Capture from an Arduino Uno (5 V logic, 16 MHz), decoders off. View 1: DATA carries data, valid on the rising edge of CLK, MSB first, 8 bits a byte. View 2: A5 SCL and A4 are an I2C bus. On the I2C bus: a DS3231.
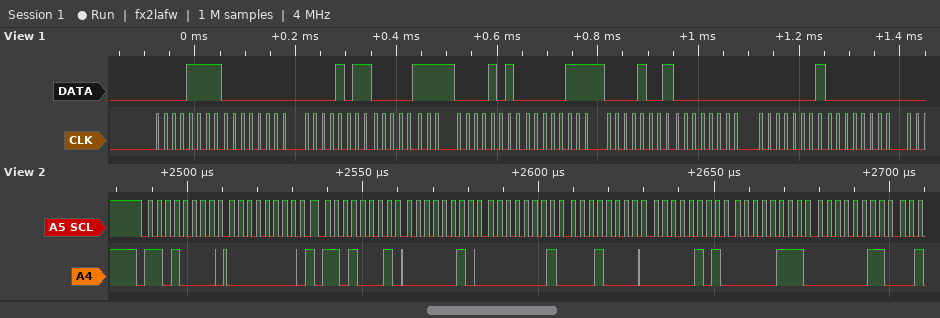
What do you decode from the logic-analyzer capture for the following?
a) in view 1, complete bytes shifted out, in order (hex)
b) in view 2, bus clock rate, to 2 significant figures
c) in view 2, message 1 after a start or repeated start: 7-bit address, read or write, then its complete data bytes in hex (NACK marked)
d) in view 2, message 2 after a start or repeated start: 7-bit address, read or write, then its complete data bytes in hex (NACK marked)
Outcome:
0x0F 0x00 0x0B 0x07 0x0A 0x07 0x09 0x00 0x01 0x00
400 kHz
0x68 write: 00
0x68 read: 02 01 10 05 07 03
